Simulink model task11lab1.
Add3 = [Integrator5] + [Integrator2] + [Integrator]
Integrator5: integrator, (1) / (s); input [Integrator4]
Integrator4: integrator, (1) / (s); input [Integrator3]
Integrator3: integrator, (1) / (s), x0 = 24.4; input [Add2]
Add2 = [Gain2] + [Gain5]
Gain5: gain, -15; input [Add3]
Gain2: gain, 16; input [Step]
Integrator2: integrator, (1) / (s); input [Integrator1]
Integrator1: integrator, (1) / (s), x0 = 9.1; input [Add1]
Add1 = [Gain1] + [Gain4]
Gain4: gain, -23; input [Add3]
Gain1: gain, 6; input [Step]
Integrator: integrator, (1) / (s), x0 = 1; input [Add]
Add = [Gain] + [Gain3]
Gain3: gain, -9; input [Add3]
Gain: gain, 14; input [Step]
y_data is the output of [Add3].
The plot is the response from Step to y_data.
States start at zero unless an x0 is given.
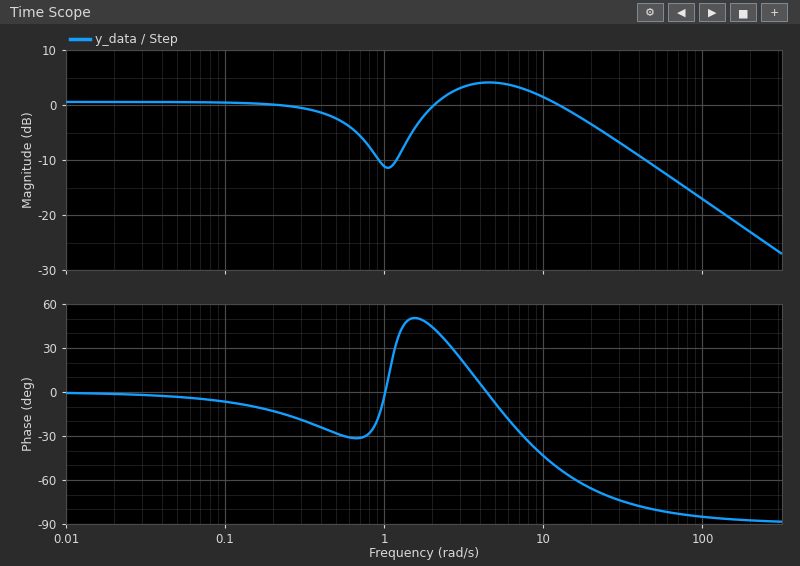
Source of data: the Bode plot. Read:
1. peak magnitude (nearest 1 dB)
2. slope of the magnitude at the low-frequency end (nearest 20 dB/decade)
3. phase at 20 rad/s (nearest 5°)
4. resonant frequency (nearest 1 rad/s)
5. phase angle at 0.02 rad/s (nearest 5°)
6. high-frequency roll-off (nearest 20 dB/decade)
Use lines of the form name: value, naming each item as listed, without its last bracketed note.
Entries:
peak magnitude: 4 dB
slope of the magnitude at the low-frequency end: 0 dB/decade
phase at 20 rad/s: -65°
resonant frequency: 5 rad/s
phase angle at 0.02 rad/s: 0°
high-frequency roll-off: -20 dB/decade
